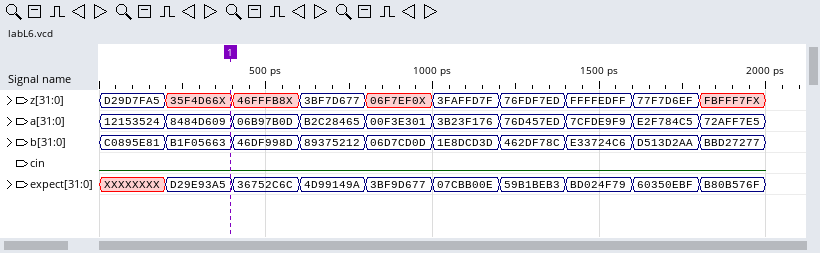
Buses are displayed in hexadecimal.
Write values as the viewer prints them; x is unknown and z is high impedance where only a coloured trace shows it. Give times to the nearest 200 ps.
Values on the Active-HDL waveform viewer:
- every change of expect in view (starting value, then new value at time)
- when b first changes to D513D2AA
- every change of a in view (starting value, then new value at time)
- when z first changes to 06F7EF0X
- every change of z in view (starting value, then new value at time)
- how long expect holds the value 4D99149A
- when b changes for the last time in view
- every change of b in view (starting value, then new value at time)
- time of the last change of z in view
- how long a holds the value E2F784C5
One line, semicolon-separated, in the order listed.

XXXXXXXX, D29E93A5 at 200 ps, 36752C6C at 400 ps, 4D99149A at 600 ps, 3BF9D677 at 800 ps, 07CBB00E at 1000 ps, 59B1BEB3 at 1200 ps, BD024F79 at 1400 ps, 60350EBF at 1600 ps, B80B576F at 1800 ps; 1600 ps; 12153524, 8484D609 at 200 ps, 06B97B0D at 400 ps, B2C28465 at 600 ps, 00F3E301 at 800 ps, 3B23F176 at 1000 ps, 76D457ED at 1200 ps, 7CFDE9F9 at 1400 ps, E2F784C5 at 1600 ps, 72AFF7E5 at 1800 ps; 800 ps; D29D7FA5, 35F4D66X at 200 ps, 46FFFB8X at 400 ps, 3BF7D677 at 600 ps, 06F7EF0X at 800 ps, 3FAFFD7F at 1000 ps, 76FDF7ED at 1200 ps, FFFFEDFF at 1400 ps, 77F7D6EF at 1600 ps, FBFFF7FX at 1800 ps; 200 ps; 1800 ps; C0895E81, B1F05663 at 200 ps, 46DF998D at 400 ps, 89375212 at 600 ps, 06D7CD0D at 800 ps, 1E8DCD3D at 1000 ps, 462DF78C at 1200 ps, E33724C6 at 1400 ps, D513D2AA at 1600 ps, BBD27277 at 1800 ps; 1800 ps; 200 ps
